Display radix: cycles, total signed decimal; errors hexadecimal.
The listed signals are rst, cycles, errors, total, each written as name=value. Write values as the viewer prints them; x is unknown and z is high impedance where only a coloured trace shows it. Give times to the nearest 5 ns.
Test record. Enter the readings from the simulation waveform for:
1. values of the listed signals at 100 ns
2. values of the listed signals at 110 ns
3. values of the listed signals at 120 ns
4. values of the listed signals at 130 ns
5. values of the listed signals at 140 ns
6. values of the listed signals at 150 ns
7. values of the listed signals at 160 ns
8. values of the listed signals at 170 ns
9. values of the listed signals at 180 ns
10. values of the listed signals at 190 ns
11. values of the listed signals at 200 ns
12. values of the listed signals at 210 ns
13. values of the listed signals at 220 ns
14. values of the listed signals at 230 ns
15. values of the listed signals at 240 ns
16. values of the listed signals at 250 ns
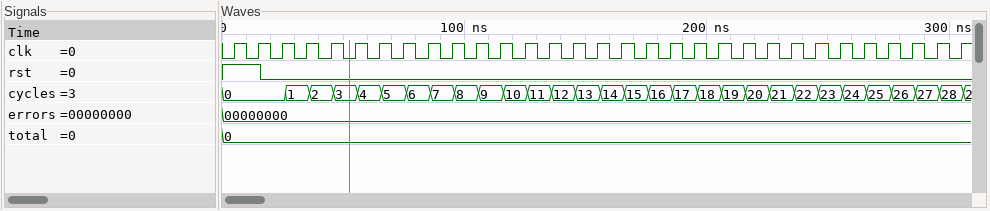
rst=0, cycles=8, errors=00000000, total=0
rst=0, cycles=9, errors=00000000, total=0
rst=0, cycles=10, errors=00000000, total=0
rst=0, cycles=11, errors=00000000, total=0
rst=0, cycles=12, errors=00000000, total=0
rst=0, cycles=13, errors=00000000, total=0
rst=0, cycles=14, errors=00000000, total=0
rst=0, cycles=15, errors=00000000, total=0
rst=0, cycles=16, errors=00000000, total=0
rst=0, cycles=17, errors=00000000, total=0
rst=0, cycles=18, errors=00000000, total=0
rst=0, cycles=19, errors=00000000, total=0
rst=0, cycles=20, errors=00000000, total=0
rst=0, cycles=21, errors=00000000, total=0
rst=0, cycles=22, errors=00000000, total=0
rst=0, cycles=23, errors=00000000, total=0
